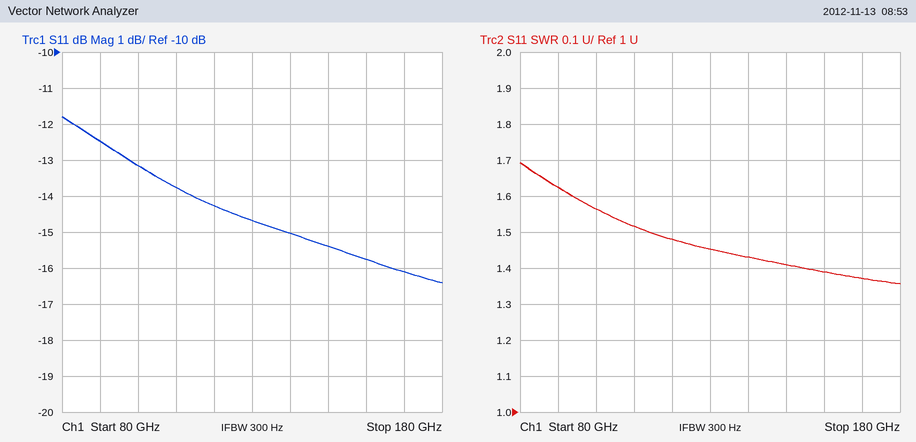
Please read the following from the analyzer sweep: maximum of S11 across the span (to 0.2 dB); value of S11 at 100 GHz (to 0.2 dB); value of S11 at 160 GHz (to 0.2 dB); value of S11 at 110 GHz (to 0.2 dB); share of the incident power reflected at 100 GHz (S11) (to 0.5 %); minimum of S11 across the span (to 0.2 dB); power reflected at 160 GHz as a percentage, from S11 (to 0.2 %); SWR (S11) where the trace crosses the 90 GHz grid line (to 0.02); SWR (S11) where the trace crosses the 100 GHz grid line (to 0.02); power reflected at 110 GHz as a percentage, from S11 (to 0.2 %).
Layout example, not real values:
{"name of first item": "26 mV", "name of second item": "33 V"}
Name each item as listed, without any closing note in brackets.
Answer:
{"maximum of S11 across the span": "-11.8 dB", "value of S11 at 100 GHz": "-13.2 dB", "value of S11 at 160 GHz": "-15.8 dB", "value of S11 at 110 GHz": "-13.8 dB", "share of the incident power reflected at 100 GHz (S11)": "5.0 %", "minimum of S11 across the span": "-16.4 dB", "power reflected at 160 GHz as a percentage, from S11": "2.6 %", "SWR (S11) where the trace crosses the 90 GHz grid line": "1.62", "SWR (S11) where the trace crosses the 100 GHz grid line": "1.56", "power reflected at 110 GHz as a percentage, from S11": "4.2 %"}
